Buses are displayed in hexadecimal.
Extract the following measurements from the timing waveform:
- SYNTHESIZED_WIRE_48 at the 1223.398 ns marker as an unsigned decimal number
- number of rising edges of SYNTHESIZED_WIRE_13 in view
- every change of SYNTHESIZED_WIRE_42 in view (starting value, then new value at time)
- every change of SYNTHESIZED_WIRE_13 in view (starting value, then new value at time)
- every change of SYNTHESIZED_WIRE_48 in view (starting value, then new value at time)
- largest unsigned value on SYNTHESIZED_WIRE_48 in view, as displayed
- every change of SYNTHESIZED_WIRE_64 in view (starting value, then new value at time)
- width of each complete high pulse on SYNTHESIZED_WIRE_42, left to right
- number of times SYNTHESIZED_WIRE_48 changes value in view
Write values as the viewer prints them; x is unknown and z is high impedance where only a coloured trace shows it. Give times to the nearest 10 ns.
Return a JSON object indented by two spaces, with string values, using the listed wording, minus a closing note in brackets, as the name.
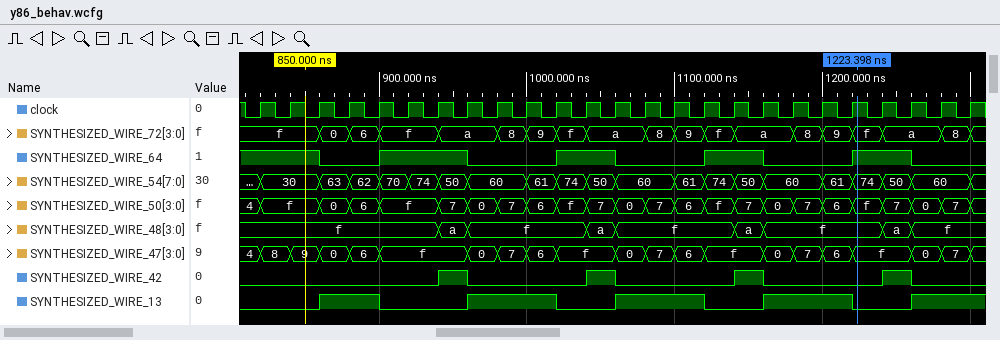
{
  "SYNTHESIZED_WIRE_48 at the 1223.398 ns marker as an unsigned decimal number": "15",
  "number of rising edges of SYNTHESIZED_WIRE_13 in view": "5",
  "every change of SYNTHESIZED_WIRE_42 in view": "0, 1 at 940 ns, 0 at 960 ns, 1 at 1040 ns, 0 at 1060 ns, 1 at 1140 ns, 0 at 1160 ns, 1 at 1240 ns, 0 at 1260 ns",
  "every change of SYNTHESIZED_WIRE_13 in view": "0, 1 at 860 ns, 0 at 900 ns, 1 at 960 ns, 0 at 1020 ns, 1 at 1060 ns, 0 at 1120 ns, 1 at 1160 ns, 0 at 1220 ns, 1 at 1260 ns",
  "every change of SYNTHESIZED_WIRE_48 in view": "f, a at 940 ns, f at 960 ns, a at 1040 ns, f at 1060 ns, a at 1140 ns, f at 1160 ns, a at 1240 ns, f at 1260 ns",
  "largest unsigned value on SYNTHESIZED_WIRE_48 in view, as displayed": "f",
  "every change of SYNTHESIZED_WIRE_64 in view": "1, 0 at 860 ns, 1 at 900 ns, 0 at 960 ns, 1 at 1020 ns, 0 at 1060 ns, 1 at 1120 ns, 0 at 1160 ns, 1 at 1220 ns, 0 at 1260 ns",
  "width of each complete high pulse on SYNTHESIZED_WIRE_42, left to right": "20 ns, 20 ns, 20 ns, 20 ns",
  "number of times SYNTHESIZED_WIRE_48 changes value in view": "8"
}
